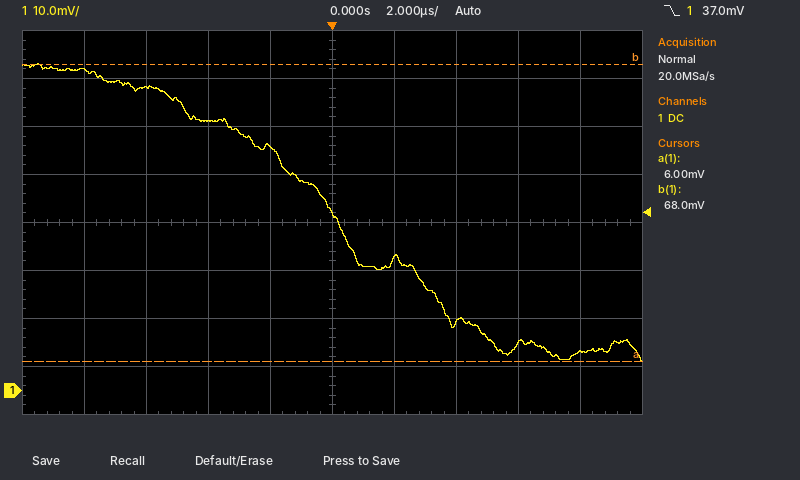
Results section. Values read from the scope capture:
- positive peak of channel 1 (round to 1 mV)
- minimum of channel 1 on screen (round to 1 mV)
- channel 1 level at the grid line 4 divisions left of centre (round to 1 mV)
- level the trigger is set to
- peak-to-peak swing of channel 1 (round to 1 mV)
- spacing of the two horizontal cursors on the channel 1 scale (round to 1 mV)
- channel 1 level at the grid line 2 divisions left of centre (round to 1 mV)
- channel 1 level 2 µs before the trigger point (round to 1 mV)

68 mV
6 mV
67 mV
37.0 mV
62 mV
62 mV
56 mV
51 mV
